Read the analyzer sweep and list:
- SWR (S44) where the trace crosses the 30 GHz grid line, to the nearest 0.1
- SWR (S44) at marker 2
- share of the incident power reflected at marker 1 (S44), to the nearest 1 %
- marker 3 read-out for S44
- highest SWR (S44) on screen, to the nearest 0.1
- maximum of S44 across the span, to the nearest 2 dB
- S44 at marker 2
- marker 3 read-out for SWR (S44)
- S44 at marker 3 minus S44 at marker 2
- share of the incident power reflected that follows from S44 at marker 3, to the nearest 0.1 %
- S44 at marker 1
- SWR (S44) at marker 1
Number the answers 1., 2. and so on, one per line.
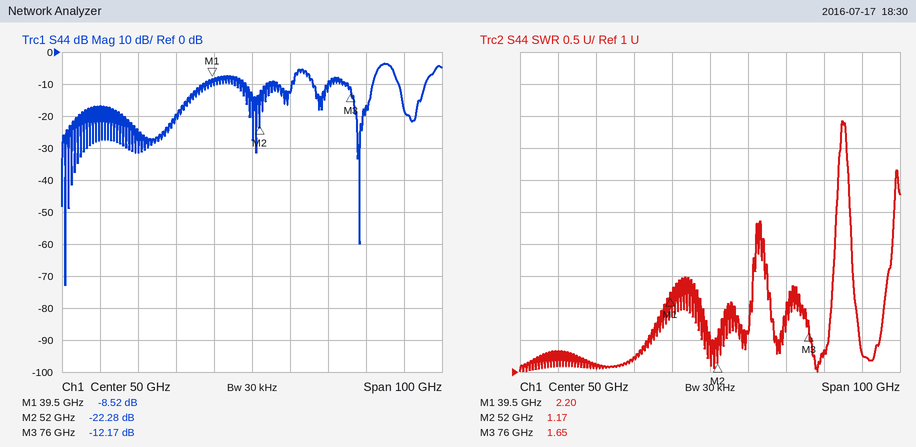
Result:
1. 1.2
2. 1.17
3. 14 %
4. -12.17 dB
5. 4.9
6. -4 dB
7. -22.28 dB
8. 1.65
9. 10.11 dB
10. 6.1 %
11. -8.52 dB
12. 2.20
